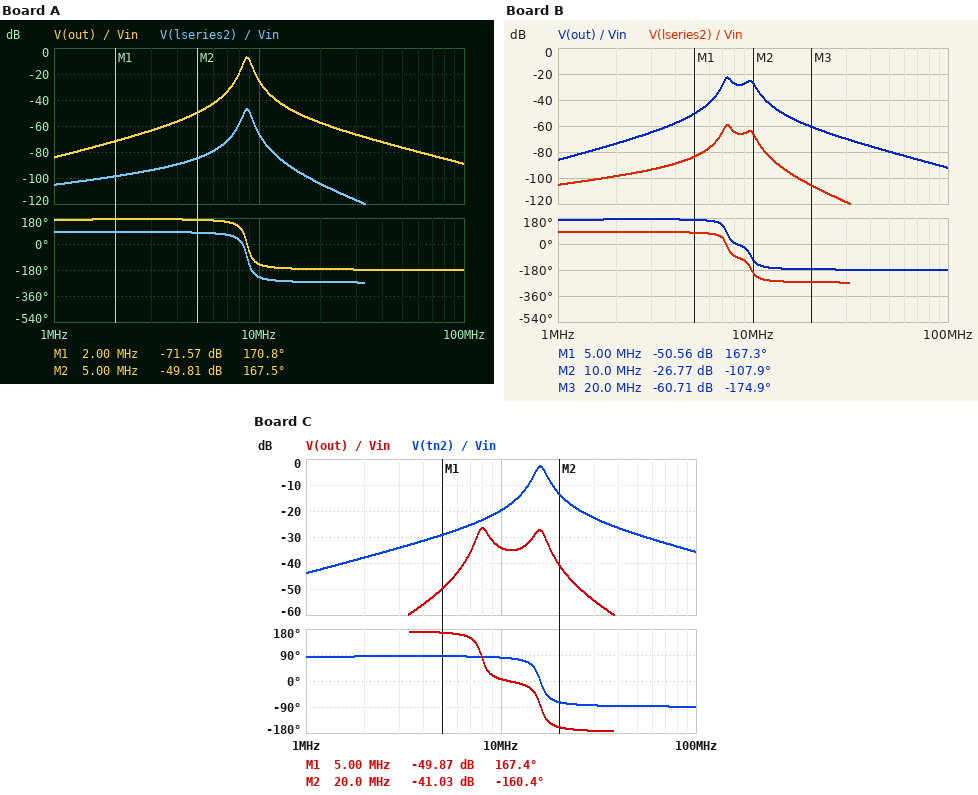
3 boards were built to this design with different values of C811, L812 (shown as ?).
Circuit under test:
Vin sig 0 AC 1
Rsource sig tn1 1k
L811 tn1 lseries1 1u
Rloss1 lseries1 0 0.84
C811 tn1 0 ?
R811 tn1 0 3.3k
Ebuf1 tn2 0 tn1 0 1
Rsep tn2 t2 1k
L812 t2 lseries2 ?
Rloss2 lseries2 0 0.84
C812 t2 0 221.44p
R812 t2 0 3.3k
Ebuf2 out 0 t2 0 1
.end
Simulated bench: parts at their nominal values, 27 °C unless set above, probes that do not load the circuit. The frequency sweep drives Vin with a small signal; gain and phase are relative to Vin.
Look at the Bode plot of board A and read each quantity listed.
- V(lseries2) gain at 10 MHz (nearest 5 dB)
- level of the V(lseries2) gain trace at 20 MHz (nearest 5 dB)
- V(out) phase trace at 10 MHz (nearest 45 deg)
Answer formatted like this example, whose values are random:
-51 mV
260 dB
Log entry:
-65 dB
-105 dB
-135 deg
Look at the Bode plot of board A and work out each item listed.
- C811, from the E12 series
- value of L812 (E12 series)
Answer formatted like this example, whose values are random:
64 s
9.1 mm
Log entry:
330 pF
1.5 µH
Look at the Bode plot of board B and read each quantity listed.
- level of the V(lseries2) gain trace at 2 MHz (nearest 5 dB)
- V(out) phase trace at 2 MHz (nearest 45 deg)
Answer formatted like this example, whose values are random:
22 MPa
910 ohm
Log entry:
-100 dB
180 deg
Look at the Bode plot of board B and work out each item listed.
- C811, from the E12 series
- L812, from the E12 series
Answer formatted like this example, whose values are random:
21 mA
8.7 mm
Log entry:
470 pF
1.2 µH
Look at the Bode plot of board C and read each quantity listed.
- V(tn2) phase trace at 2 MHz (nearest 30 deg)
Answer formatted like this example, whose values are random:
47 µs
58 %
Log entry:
90 deg
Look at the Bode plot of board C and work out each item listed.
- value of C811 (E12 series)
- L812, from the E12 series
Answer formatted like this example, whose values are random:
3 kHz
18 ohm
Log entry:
100 pF
1.8 µH
